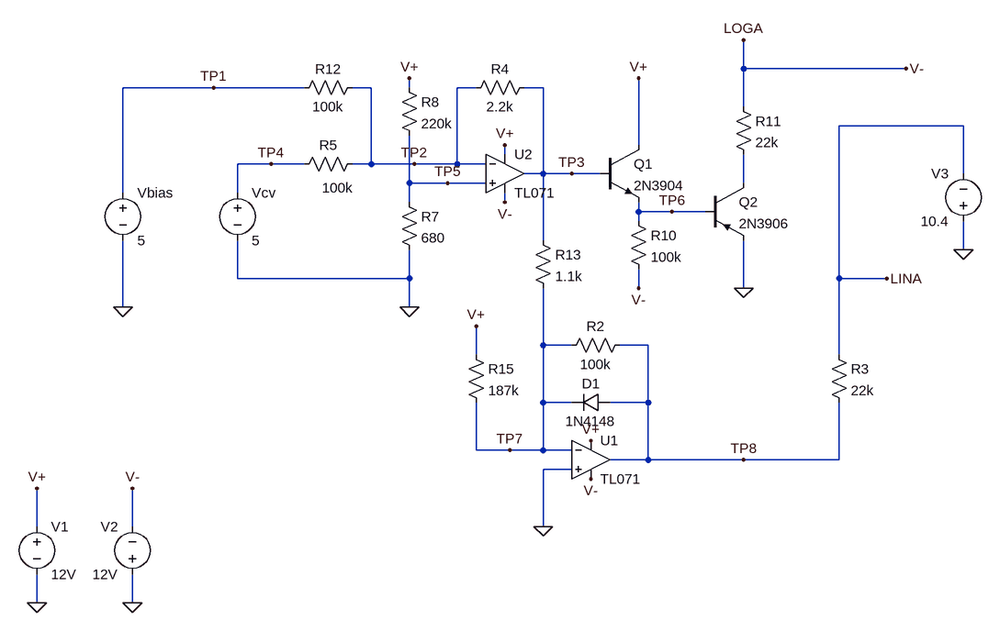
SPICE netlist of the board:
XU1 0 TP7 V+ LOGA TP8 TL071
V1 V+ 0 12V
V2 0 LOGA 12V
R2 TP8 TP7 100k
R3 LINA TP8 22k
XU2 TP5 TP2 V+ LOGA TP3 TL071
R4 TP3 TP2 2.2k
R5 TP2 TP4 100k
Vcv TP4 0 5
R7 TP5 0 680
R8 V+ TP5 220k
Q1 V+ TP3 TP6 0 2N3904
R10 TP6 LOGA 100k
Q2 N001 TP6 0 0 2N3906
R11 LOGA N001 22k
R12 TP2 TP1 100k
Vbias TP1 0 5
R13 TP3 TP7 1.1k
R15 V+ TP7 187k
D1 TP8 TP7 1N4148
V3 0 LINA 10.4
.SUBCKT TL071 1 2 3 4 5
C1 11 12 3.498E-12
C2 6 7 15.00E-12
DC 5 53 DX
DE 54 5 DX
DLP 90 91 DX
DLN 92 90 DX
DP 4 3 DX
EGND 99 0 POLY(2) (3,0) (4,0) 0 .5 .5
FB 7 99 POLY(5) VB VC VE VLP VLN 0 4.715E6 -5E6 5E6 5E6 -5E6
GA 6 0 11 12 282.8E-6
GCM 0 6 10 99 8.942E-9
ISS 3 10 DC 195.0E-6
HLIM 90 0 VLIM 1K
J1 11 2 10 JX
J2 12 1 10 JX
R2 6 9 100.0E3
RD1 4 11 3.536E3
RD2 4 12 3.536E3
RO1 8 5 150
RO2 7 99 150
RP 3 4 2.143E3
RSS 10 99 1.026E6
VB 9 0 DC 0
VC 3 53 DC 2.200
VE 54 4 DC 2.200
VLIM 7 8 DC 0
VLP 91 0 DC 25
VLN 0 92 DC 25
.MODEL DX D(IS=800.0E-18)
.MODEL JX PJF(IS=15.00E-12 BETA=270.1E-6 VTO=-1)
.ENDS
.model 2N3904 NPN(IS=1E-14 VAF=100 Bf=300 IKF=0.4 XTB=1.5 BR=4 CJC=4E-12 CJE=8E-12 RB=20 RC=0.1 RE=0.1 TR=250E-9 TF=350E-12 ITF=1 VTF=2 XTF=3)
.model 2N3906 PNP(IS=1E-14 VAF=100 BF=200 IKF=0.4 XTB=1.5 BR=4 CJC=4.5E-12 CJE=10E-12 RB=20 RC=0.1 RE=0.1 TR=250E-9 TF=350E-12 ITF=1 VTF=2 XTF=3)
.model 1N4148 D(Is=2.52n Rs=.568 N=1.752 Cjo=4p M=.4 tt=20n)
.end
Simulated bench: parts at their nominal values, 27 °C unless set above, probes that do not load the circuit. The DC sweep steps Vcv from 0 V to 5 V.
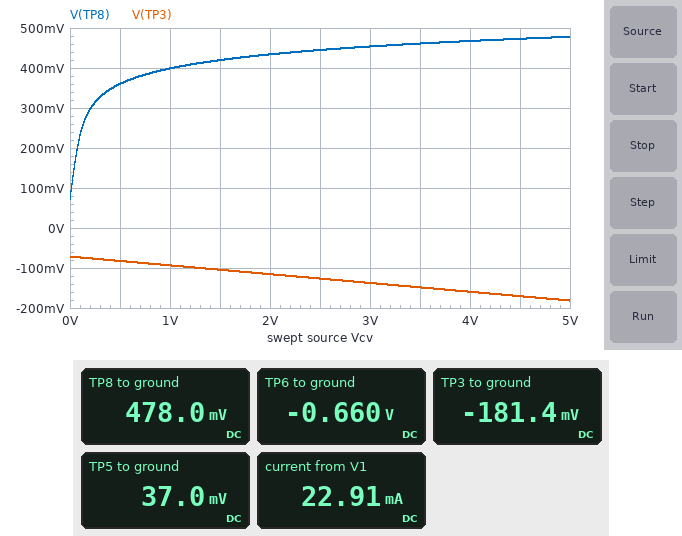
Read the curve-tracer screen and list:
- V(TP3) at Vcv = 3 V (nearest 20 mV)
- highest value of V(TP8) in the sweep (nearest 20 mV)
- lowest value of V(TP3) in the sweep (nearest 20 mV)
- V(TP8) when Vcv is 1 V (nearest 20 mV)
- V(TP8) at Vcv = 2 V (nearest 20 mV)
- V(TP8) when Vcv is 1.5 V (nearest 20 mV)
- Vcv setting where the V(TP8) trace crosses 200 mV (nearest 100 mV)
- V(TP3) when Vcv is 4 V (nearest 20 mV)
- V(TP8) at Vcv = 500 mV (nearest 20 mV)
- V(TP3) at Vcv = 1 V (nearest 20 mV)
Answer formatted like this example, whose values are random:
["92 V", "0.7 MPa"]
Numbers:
["-140 mV", "480 mV", "-180 mV", "400 mV", "440 mV", "420 mV", "100 mV", "-160 mV", "360 mV", "-100 mV"]
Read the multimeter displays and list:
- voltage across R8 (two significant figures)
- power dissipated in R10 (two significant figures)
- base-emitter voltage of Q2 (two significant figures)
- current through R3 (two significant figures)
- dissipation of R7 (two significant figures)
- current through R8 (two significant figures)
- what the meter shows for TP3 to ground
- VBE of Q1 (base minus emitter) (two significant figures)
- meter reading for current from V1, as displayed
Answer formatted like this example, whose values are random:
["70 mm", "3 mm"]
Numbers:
["12 V", "1.3 mW", "-660 mV", "490 µA", "2.0 µW", "54 µA", "-181.4 mV", "480 mV", "22.91 mA"]
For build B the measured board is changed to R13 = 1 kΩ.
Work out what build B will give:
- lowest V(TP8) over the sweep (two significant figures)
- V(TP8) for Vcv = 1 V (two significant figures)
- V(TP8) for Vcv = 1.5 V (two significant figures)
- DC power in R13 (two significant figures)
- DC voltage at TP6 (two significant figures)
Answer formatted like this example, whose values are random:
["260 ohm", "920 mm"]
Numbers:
["330 mV", "420 mV", "430 mV", "33 µW", "-660 mV"]
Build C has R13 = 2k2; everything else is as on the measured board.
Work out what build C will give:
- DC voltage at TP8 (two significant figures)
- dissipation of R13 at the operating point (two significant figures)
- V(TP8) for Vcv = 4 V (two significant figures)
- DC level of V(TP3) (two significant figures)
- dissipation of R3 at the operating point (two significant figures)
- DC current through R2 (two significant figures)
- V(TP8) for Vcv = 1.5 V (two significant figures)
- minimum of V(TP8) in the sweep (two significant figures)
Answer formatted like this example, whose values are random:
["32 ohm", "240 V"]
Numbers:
["390 mV", "15 µW", "340 mV", "-180 mV", "5.3 mW", "3.9 µA", "-1.7 V", "-3.2 V"]
